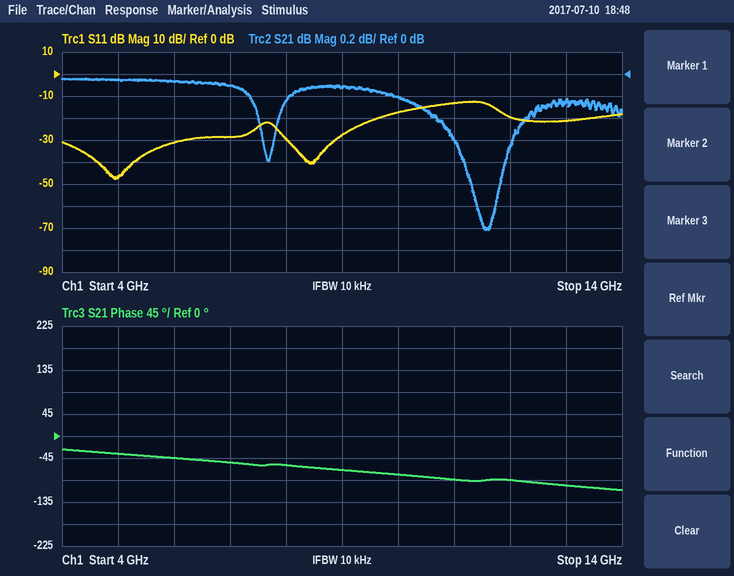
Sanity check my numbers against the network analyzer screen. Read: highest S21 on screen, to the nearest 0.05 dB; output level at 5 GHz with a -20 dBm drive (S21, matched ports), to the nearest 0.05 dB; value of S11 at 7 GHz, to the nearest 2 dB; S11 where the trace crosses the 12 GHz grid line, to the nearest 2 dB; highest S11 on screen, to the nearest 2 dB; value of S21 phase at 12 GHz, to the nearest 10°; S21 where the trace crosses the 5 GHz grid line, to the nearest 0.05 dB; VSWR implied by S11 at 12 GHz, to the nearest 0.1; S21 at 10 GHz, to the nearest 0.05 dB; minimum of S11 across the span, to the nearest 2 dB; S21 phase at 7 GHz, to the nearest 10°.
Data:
-0.05 dB
-20.05 dBm
-28 dB
-20 dB
-12 dB
-90°
-0.05 dB
1.2
-0.20 dB
-48 dB
-50°
